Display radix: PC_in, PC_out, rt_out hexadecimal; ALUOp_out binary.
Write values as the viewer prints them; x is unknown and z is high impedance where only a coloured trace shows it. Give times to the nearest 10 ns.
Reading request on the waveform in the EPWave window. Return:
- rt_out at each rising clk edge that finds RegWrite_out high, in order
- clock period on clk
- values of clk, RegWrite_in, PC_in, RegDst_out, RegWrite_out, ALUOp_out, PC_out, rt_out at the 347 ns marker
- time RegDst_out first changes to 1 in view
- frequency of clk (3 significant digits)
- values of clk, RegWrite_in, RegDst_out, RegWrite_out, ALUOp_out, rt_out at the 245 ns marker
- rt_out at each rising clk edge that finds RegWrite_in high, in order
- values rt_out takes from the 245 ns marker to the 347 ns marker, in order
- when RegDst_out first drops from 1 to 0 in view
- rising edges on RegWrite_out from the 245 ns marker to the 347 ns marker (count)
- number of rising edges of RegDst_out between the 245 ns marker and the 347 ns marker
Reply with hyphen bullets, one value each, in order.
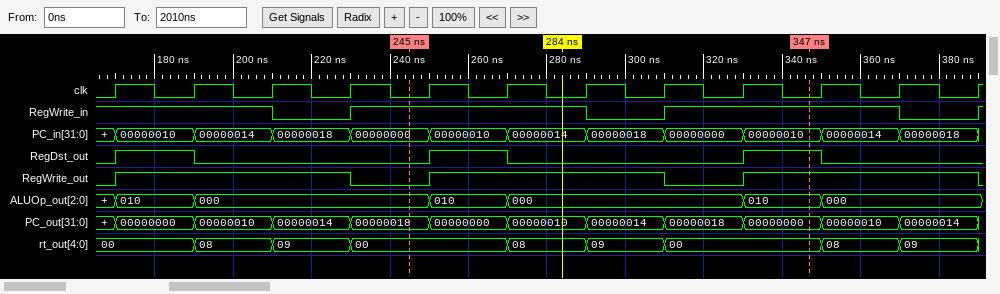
- 00, 08, 09, 00, 08, 09, 00, 08, 09
- 20 ns
- clk=0, RegWrite_in=1, PC_in=00000010, RegDst_out=1, RegWrite_out=1, ALUOp_out=010, PC_out=00000000, rt_out=00
- 170 ns
- 50.0 MHz
- clk=0, RegWrite_in=1, RegDst_out=0, RegWrite_out=0, ALUOp_out=000, rt_out=00
- 00, 00, 08, 00, 00, 08, 00, 00, 08
- 00, 08, 09, 00
- 190 ns
- 2
- 2
